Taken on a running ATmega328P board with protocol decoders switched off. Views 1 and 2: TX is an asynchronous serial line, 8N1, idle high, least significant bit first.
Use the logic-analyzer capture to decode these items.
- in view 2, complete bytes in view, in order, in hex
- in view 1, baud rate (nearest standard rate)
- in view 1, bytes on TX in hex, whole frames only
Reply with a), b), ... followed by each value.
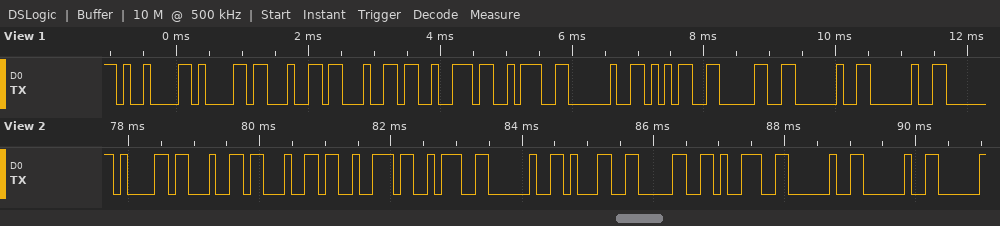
a) 61 64 64 72 3A 20 31 30 39 20 20
b) 9600 baud
c) 09 61 64 64 72 3A 20 35 30 20 20
